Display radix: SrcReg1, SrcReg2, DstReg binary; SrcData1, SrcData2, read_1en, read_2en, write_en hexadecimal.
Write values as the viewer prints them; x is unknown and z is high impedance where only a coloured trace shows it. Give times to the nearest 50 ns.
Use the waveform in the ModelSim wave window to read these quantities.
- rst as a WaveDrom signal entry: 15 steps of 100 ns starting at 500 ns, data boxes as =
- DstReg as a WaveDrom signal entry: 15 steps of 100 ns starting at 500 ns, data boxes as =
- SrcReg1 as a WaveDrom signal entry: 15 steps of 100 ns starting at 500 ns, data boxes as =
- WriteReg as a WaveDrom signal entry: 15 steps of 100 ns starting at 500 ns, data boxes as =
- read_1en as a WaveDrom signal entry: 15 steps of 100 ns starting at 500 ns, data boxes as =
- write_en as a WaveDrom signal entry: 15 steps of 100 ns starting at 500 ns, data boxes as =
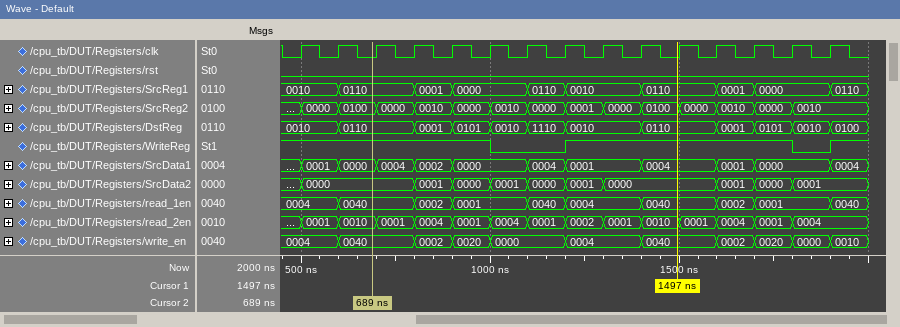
{name: 'rst', wave: '0..............'}
{name: 'DstReg', wave: '==.=====.=.====', data: '0010 0110 0001 0101 0010 1110 0010 0110 0001 0101 0010 0100'}
{name: 'SrcReg1', wave: '==.==.==.=.==.=', data: '0010 0110 0001 0000 0110 0010 0110 0001 0000 0110'}
{name: 'WriteReg', wave: '1....0.1.....01'}
{name: 'read_1en', wave: '==.==.==.=.==.=', data: '0004 0040 0002 0001 0040 0004 0040 0002 0001 0040'}
{name: 'write_en', wave: '==.===.=.=.====', data: '0004 0040 0002 0020 0000 0004 0040 0002 0020 0000 0010'}
